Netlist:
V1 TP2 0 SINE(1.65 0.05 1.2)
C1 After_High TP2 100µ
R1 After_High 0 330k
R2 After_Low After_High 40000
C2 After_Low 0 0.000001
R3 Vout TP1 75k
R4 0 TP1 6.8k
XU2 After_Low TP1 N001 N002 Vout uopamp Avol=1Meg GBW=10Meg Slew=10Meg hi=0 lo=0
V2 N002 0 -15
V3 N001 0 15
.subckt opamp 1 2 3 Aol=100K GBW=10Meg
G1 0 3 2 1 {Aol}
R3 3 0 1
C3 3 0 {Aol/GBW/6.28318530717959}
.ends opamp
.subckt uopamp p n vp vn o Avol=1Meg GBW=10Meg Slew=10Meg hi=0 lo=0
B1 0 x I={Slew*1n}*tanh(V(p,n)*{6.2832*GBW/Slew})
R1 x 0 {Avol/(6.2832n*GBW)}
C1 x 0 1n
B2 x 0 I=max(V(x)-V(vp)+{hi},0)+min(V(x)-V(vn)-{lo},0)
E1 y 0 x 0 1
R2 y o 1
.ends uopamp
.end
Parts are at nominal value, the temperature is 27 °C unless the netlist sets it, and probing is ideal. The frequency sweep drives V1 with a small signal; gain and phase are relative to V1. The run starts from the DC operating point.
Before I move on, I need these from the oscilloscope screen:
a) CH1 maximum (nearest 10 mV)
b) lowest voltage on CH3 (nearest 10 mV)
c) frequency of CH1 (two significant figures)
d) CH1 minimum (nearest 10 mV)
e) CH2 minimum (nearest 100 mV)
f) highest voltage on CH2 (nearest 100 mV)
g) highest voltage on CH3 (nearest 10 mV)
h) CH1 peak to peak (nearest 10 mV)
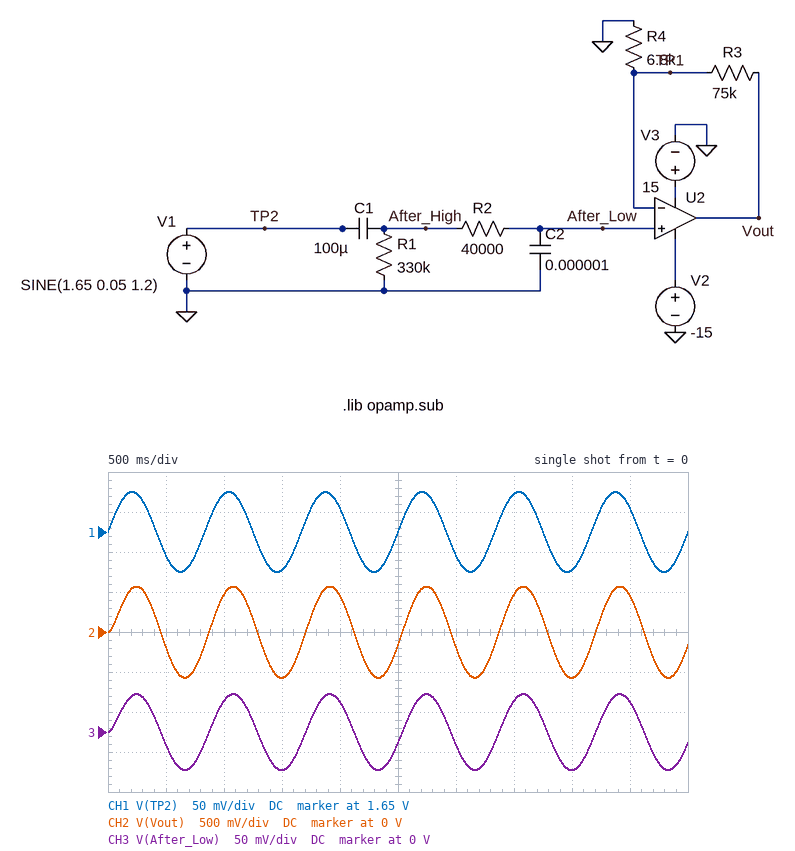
1.70 V
-50 mV
1.2 Hz
1.60 V
-600 mV
600 mV
50 mV
100 mV
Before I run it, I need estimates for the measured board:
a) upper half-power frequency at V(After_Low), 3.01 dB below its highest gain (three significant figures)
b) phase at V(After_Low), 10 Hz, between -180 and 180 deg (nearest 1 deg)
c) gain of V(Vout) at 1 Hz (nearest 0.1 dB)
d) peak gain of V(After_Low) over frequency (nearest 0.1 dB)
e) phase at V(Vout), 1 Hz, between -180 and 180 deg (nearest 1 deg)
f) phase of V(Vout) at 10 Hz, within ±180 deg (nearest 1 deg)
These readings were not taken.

4.03 Hz
-68 deg
21.3 dB
-0.1 dB
-14 deg
-68 deg
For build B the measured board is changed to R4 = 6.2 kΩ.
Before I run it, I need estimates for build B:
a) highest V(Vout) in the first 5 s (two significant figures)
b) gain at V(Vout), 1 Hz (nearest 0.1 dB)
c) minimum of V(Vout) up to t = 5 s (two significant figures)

620 mV
22.0 dB
-620 mV
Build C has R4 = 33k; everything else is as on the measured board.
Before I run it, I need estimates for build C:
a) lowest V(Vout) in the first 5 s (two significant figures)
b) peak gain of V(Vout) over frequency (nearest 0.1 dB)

-160 mV
10.2 dB
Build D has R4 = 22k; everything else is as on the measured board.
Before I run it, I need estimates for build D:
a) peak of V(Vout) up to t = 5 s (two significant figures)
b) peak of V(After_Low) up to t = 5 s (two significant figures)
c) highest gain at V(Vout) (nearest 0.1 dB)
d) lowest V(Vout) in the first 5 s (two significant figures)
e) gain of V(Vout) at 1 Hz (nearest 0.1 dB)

210 mV
47 mV
12.8 dB
-210 mV
12.5 dB
